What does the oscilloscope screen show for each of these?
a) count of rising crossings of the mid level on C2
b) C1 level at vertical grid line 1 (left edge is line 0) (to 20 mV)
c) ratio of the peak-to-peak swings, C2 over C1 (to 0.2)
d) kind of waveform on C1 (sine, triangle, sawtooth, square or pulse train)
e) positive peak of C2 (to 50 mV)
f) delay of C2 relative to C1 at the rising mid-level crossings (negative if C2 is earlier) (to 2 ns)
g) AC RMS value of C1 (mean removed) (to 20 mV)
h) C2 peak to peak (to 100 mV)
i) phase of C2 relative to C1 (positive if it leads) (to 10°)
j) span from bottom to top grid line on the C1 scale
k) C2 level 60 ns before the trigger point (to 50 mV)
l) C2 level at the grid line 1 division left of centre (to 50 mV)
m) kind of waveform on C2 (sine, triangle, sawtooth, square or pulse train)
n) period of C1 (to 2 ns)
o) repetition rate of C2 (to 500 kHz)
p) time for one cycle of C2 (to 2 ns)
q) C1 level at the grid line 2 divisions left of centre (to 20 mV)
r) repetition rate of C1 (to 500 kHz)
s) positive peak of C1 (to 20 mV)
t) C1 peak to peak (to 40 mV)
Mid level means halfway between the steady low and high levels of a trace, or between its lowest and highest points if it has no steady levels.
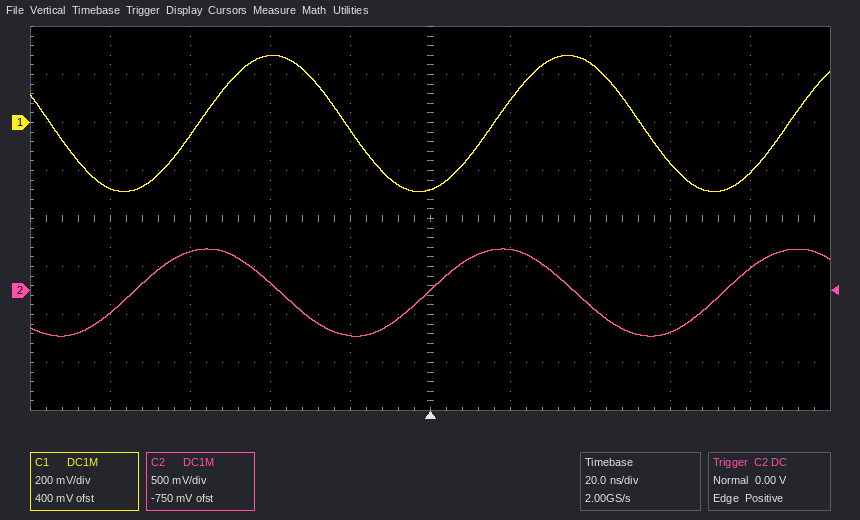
3
-280 mV
1.6
sine
450 mV
-16 ns
200 mV
900 mV
+80°
1.6 V
400 mV
-450 mV
sine
74 ns
13.5 MHz
74 ns
280 mV
13.5 MHz
280 mV
560 mV
